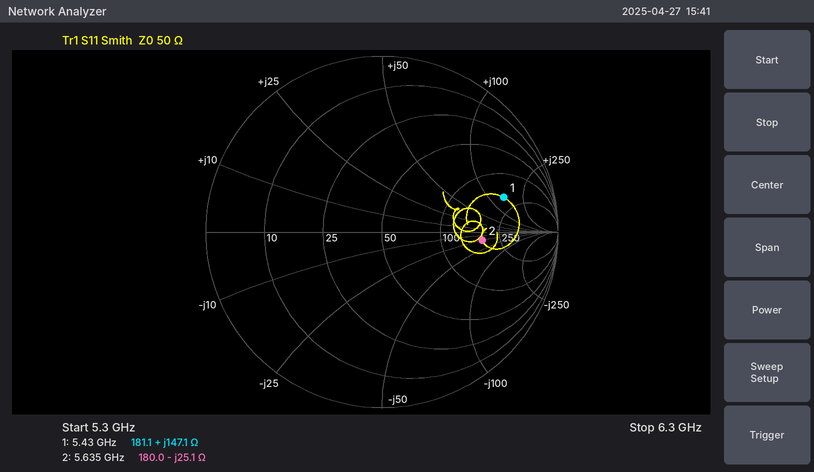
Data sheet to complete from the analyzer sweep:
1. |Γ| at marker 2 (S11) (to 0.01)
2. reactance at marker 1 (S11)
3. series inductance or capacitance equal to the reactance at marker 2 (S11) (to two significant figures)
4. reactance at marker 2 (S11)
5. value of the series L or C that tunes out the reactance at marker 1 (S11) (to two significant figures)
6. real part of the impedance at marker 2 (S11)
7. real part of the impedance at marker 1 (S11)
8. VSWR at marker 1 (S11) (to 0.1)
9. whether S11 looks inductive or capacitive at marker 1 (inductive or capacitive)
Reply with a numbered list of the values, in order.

1. 0.57
2. +147.1 Ω
3. 1.1 pF
4. -25.1 Ω
5. 200 fF
6. 180.0 Ω
7. 181.1 Ω
8. 6.1
9. inductive
